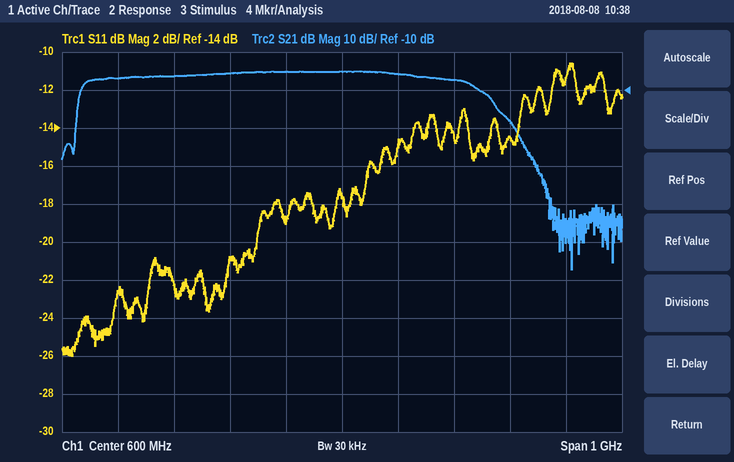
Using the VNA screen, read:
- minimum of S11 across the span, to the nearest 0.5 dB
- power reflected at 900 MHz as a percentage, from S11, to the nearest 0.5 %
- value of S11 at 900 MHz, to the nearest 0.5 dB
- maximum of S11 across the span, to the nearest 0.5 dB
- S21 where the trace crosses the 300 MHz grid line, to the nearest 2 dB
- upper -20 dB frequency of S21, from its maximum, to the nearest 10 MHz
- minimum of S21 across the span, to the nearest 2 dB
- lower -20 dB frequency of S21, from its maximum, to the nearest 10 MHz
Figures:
-26.0 dB
3.5 %
-14.5 dB
-10.5 dB
-6 dB
930 MHz
-58 dB
120 MHz
